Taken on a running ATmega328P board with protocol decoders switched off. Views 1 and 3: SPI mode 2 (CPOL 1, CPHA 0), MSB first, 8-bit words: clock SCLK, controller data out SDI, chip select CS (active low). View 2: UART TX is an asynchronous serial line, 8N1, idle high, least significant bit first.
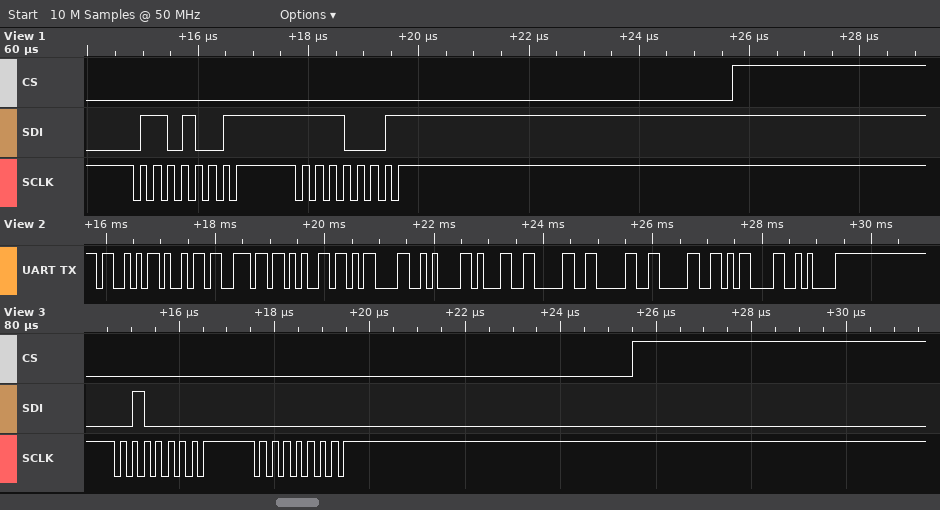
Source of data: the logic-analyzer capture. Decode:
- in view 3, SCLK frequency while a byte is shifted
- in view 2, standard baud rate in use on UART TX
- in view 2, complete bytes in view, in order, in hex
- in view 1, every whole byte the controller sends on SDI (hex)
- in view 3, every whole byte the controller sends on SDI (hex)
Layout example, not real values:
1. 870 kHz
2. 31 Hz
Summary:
1. 4 MHz
2. 9600 baud
3. 53 69 6E 65 0D 0A 31 30 30 30 0D 0A
4. 69 F1
5. 0x20 0x00
